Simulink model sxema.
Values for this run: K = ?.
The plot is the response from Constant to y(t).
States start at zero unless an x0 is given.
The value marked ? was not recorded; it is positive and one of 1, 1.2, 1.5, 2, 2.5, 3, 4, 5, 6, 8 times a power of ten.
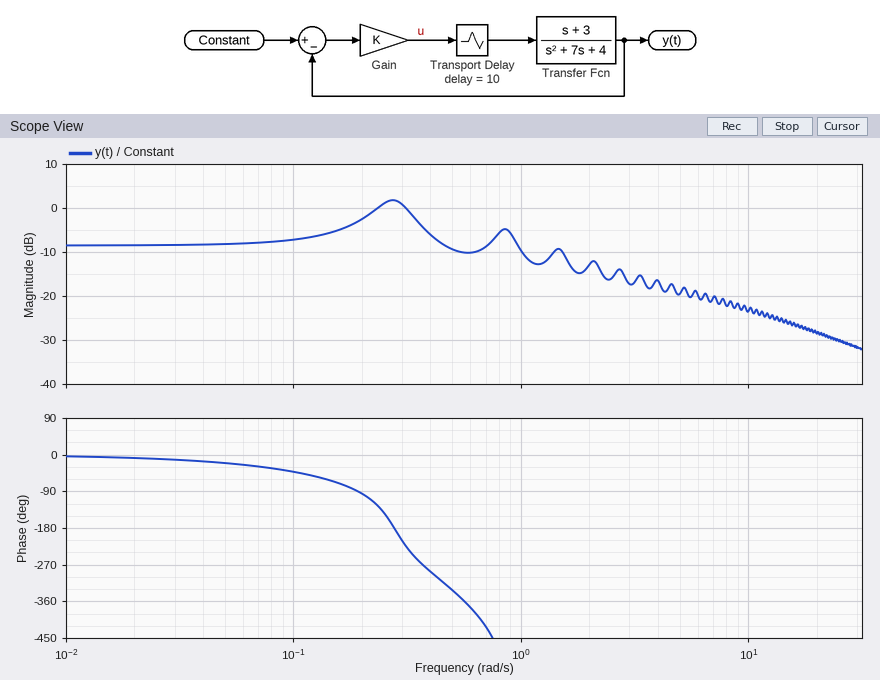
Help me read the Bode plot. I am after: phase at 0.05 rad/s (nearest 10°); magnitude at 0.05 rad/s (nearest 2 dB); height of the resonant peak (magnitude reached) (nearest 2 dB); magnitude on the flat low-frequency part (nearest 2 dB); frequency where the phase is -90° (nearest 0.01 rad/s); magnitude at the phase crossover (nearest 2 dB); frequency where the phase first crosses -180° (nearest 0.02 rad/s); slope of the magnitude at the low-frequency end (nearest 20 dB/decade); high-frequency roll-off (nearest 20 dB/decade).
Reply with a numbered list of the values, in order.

1. -20°
2. -8 dB
3. 2 dB
4. -8 dB
5. 0.19 rad/s
6. 2 dB
7. 0.28 rad/s
8. 0 dB/decade
9. -20 dB/decade
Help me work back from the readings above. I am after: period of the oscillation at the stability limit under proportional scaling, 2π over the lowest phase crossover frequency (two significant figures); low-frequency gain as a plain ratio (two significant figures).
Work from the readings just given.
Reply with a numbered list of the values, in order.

1. 22 s
2. 0.40
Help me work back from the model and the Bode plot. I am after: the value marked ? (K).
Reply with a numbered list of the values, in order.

1. 0.8
